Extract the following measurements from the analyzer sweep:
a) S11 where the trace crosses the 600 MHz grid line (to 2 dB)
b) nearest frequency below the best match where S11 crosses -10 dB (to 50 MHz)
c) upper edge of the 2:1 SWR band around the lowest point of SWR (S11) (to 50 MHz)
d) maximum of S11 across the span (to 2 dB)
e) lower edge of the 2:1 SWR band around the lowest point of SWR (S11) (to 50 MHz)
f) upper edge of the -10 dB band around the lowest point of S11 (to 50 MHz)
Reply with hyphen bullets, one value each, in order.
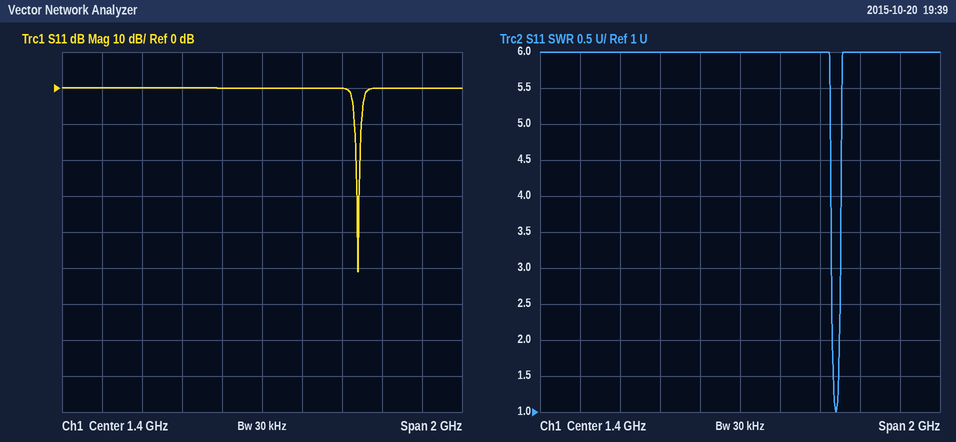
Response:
- 0 dB
- 1.85 GHz
- 1.90 GHz
- 0 dB
- 1.85 GHz
- 1.90 GHz
